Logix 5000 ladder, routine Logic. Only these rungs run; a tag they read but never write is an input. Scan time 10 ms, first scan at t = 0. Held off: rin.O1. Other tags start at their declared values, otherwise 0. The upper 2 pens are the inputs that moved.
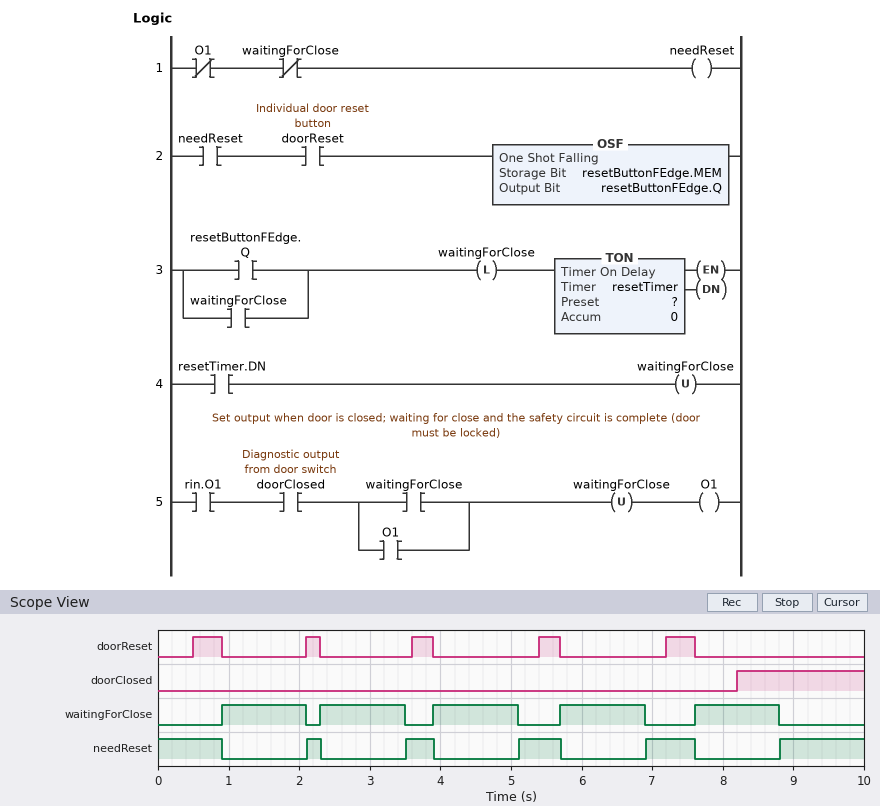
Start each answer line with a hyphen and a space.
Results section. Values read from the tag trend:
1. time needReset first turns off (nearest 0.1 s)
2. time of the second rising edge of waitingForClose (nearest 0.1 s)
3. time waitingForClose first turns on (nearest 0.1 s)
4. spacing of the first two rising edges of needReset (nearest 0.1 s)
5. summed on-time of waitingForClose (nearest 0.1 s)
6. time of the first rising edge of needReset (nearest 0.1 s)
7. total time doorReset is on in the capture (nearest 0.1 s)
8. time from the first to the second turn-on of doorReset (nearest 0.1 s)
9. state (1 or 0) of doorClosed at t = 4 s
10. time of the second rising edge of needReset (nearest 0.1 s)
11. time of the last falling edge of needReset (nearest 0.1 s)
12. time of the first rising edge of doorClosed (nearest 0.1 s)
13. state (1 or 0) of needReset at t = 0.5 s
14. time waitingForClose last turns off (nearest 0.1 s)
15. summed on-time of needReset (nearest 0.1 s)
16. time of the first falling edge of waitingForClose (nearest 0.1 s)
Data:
- 0.9 s
- 2.3 s
- 0.9 s
- 1.4 s
- 6.0 s
- 2.1 s
- 1.6 s
- 1.6 s
- 0
- 3.5 s
- 7.6 s
- 8.2 s
- 1
- 8.8 s
- 4.0 s
- 2.1 s
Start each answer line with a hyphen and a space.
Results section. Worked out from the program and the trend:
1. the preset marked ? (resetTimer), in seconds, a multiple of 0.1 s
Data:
- 1.2 s
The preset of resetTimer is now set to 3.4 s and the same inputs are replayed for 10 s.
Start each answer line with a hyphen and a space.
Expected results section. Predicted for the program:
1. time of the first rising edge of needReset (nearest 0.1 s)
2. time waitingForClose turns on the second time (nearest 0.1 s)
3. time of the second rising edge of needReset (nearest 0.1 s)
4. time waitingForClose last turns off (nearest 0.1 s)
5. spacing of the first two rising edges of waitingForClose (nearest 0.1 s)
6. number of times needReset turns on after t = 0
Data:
- 4.3 s
- 5.7 s
- 9.1 s
- 9.1 s
- 4.8 s
- 2
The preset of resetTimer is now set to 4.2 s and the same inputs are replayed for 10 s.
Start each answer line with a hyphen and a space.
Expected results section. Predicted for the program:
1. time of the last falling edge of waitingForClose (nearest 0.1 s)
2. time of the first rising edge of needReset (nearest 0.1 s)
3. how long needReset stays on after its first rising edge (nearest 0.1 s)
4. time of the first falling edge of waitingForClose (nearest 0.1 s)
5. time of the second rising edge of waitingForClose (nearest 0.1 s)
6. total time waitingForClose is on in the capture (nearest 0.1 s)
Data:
- 9.9 s
- 5.1 s
- 0.6 s
- 5.1 s
- 5.7 s
- 8.4 s
